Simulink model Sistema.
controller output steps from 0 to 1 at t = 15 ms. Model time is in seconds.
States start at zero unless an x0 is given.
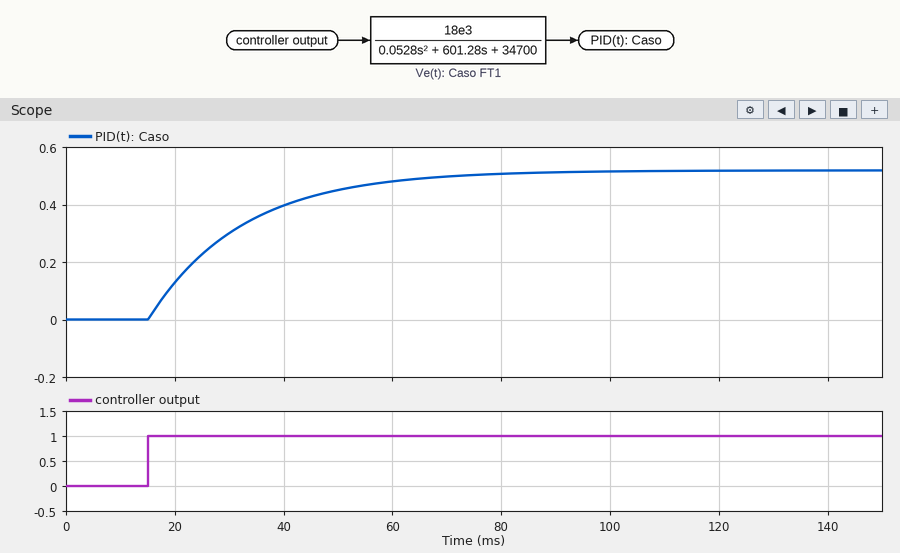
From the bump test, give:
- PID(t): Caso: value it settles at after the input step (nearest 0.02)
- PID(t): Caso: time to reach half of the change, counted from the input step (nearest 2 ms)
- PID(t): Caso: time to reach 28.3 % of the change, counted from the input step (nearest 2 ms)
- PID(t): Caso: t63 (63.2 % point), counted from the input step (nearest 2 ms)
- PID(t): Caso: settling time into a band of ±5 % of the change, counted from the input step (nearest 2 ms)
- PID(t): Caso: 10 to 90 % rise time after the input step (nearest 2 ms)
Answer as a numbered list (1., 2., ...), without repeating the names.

1. 0.52
2. 12 ms
3. 6 ms
4. 18 ms
5. 52 ms
6. 38 ms
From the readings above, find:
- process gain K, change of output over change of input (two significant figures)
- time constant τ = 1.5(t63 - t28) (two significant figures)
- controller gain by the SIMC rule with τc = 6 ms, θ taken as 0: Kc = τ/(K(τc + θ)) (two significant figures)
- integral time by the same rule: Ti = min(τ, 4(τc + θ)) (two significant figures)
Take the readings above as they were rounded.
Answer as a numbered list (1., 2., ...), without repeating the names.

1. 0.52
2. 18 ms
3. 5.8
4. 18 ms
